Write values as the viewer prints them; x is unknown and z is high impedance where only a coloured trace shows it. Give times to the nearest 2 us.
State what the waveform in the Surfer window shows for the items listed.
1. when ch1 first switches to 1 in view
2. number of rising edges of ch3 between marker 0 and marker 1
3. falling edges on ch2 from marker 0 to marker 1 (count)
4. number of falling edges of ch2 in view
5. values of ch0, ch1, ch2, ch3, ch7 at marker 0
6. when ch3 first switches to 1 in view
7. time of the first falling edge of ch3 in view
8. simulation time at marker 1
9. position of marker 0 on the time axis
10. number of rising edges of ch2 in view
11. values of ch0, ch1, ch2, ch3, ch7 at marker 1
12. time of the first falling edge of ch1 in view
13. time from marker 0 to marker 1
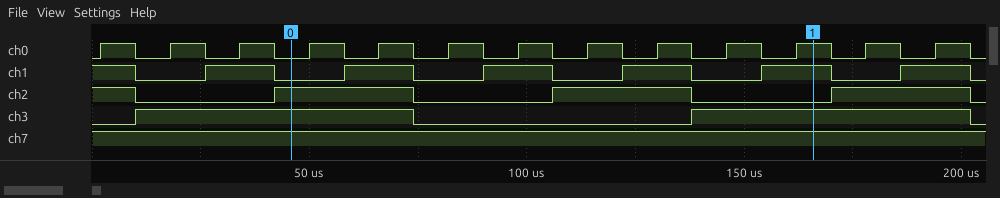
26 us
1
2
4
ch0=0, ch1=0, ch2=1, ch3=1, ch7=1
10 us
74 us
166 us
46 us
3
ch0=1, ch1=1, ch2=0, ch3=1, ch7=1
10 us
120 us
